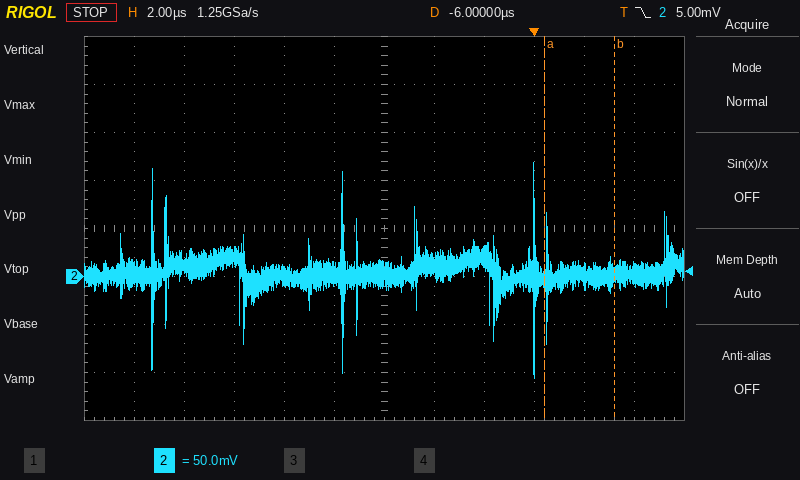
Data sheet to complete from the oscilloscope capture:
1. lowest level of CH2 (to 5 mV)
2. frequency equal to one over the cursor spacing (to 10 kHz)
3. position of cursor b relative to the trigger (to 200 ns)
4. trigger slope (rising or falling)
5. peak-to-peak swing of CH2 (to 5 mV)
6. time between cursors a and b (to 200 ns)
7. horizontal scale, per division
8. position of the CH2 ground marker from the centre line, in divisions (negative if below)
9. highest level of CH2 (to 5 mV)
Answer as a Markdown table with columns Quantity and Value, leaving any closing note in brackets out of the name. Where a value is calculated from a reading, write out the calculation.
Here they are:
| Quantity | Value |
|---|---|
| lowest level of CH2 | -105 mV |
| frequency equal to one over the cursor spacing | 1 / 2.8 µs ≈ 360 kHz |
| position of cursor b relative to the trigger | +3.2 µs |
| trigger slope | falling |
| peak-to-peak swing of CH2 | 120 mV − (-105 mV) = 225 mV |
| time between cursors a and b | 2.8 µs |
| horizontal scale, per division | 2 µs |
| position of the CH2 ground marker from the centre line, in divisions | -1.0 div |
| highest level of CH2 | 120 mV |
